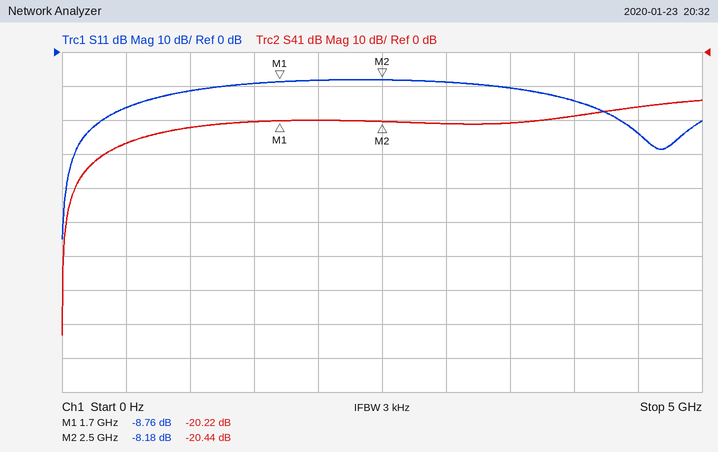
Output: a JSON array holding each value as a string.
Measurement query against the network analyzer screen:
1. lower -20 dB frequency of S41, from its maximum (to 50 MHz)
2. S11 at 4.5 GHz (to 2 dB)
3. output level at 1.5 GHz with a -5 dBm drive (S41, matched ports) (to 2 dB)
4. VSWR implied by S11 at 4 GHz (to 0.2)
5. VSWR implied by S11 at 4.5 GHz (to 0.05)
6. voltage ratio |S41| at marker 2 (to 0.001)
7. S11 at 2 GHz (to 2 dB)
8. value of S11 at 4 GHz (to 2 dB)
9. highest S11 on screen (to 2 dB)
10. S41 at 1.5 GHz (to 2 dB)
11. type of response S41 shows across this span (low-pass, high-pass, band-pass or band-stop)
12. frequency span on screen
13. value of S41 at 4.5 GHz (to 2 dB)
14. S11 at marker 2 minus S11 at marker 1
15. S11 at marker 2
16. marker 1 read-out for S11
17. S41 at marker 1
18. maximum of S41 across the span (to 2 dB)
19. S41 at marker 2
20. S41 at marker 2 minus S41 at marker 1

["200 MHz", "-24 dB", "-26 dBm", "1.4", "1.15", "0.095", "-8 dB", "-14 dB", "-8 dB", "-20 dB", "high-pass", "5 GHz", "-16 dB", "0.58 dB", "-8.18 dB", "-8.76 dB", "-20.22 dB", "-14 dB", "-20.44 dB", "-0.22 dB"]
